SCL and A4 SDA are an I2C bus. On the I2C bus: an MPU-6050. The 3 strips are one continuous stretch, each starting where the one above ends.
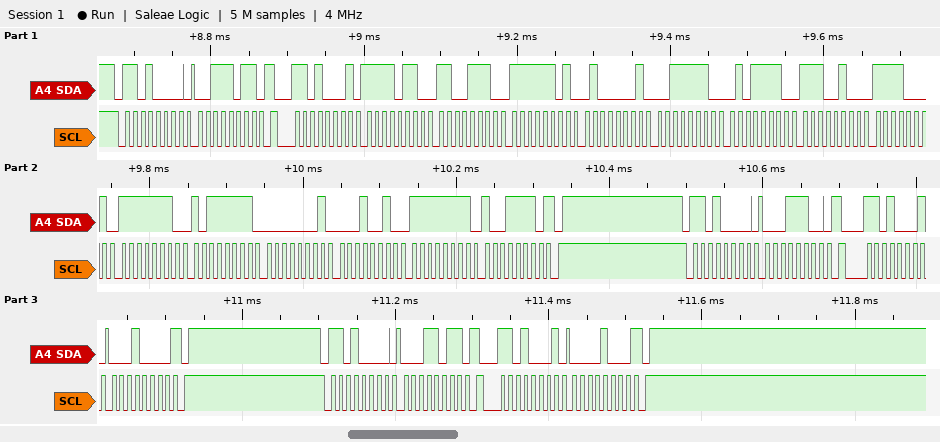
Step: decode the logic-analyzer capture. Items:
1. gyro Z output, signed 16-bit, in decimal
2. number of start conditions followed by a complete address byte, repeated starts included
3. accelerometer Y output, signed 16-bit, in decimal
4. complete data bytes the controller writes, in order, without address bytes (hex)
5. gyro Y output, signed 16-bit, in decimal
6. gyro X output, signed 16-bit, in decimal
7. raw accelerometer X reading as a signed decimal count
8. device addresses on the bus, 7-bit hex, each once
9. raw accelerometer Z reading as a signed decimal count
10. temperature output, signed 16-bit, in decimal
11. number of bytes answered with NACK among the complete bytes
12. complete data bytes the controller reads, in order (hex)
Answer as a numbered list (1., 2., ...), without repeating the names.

1. -98
2. 6
3. -703
4. 3B 1C 1B
5. 274
6. -321
7. -2354
8. 0x68
9. 15966
10. -6927
11. 3
12. F6 CE FD 41 3E 5E E4 F1 FE BF 01 12 FF 9E 10 08
